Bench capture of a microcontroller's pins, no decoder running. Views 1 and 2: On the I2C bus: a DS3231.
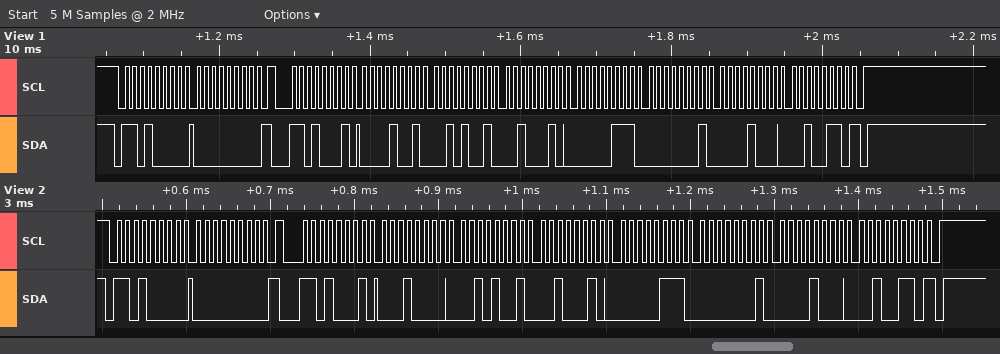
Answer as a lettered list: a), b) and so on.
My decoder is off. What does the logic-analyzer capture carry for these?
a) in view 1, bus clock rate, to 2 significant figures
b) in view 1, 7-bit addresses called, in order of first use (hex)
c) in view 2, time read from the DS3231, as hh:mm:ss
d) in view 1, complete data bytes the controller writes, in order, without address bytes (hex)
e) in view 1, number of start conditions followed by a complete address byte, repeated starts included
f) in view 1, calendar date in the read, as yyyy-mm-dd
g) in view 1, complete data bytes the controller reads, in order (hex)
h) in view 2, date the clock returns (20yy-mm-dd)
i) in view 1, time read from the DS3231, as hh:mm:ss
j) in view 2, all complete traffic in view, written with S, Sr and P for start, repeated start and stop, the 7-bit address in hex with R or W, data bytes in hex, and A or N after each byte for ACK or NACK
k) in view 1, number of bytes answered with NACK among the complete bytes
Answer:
a) 100 kHz
b) 0x68
c) 22:29:10
d) 00
e) 2
f) 2026-08-01
g) 09 29 22 07 01 08 26
h) 2026-08-01
i) 22:29:09
j) S 68W A 00 A Sr 68R A 10 A 29 A 22 A 07 A 01 A 08 A 26 N P
k) 1
